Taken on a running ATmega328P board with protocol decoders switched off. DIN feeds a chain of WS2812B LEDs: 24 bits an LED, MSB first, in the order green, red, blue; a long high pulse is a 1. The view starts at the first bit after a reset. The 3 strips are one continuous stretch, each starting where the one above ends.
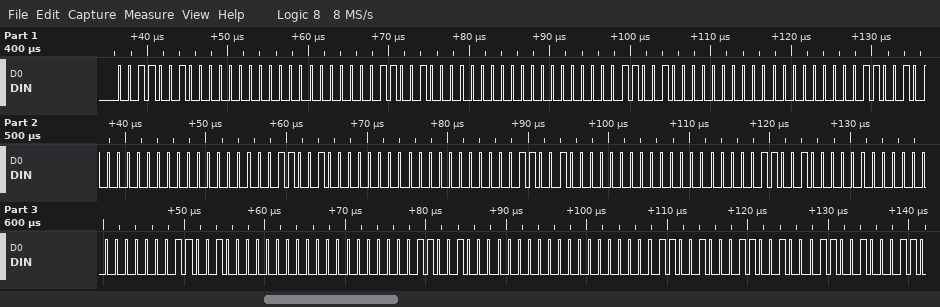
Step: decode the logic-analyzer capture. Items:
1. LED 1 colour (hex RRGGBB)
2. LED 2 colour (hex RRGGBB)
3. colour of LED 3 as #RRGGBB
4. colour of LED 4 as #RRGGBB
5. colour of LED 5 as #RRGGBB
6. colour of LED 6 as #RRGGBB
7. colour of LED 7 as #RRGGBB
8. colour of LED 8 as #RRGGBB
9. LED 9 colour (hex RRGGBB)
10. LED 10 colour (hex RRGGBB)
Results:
#003200
#003200
#003200
#003200
#003200
#003200
#003200
#003200
#003200
#323232
